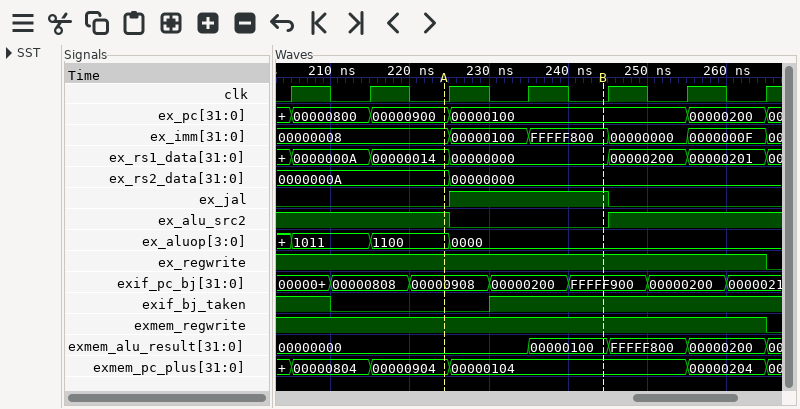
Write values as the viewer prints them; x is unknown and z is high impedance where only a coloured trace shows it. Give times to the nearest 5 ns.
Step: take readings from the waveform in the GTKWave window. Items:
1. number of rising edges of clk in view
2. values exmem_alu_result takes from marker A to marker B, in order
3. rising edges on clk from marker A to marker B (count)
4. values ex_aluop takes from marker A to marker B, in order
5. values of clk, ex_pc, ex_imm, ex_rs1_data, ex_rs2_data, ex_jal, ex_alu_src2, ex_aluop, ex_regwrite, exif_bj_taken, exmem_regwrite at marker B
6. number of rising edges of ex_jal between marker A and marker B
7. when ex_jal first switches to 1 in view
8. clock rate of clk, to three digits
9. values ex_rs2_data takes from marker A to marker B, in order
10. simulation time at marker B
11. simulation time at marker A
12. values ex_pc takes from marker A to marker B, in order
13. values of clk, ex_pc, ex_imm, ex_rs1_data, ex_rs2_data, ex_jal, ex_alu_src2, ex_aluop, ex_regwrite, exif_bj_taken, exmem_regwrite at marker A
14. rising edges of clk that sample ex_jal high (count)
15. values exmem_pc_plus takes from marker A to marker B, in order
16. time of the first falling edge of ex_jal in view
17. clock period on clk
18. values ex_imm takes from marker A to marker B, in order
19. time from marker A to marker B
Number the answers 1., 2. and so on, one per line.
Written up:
1. 7
2. 00000000, 00000100
3. 2
4. 1100, 0000
5. clk=0, ex_pc=00000100, ex_imm=FFFFF800, ex_rs1_data=00000000, ex_rs2_data=00000000, ex_jal=1, ex_alu_src2=0, ex_aluop=0000, ex_regwrite=1, exif_bj_taken=1, exmem_regwrite=1
6. 1
7. 225 ns
8. 100 MHz
9. 0000000A, 00000000
10. 245 ns
11. 225 ns
12. 00000900, 00000100
13. clk=0, ex_pc=00000900, ex_imm=00000008, ex_rs1_data=00000014, ex_rs2_data=0000000A, ex_jal=0, ex_alu_src2=1, ex_aluop=1100, ex_regwrite=1, exif_bj_taken=0, exmem_regwrite=1
14. 2
15. 00000904, 00000104
16. 245 ns
17. 10 ns
18. 00000008, 00000100, FFFFF800
19. 20 ns
